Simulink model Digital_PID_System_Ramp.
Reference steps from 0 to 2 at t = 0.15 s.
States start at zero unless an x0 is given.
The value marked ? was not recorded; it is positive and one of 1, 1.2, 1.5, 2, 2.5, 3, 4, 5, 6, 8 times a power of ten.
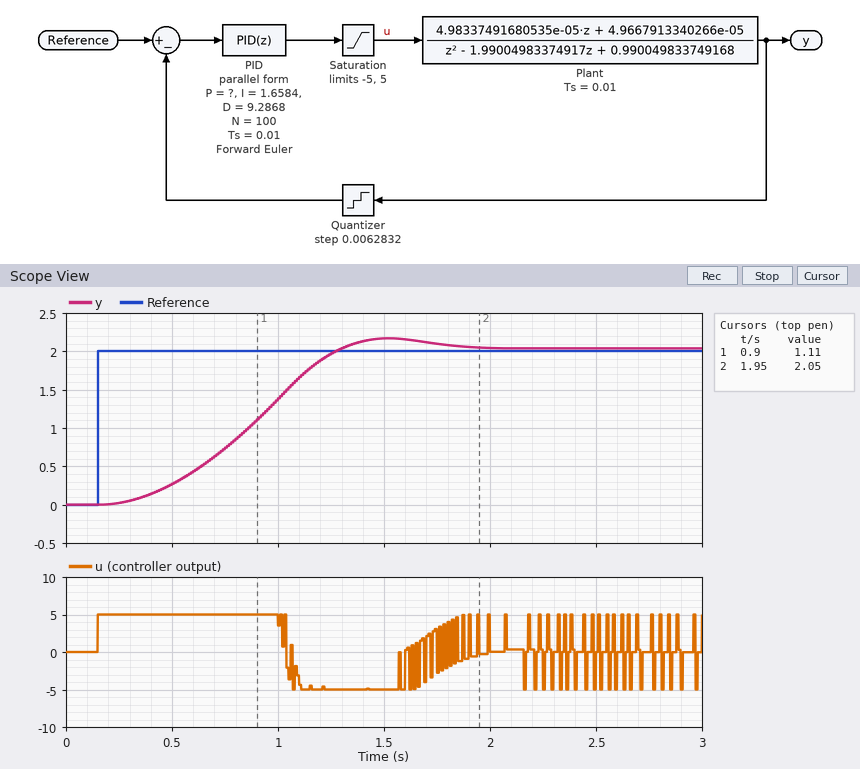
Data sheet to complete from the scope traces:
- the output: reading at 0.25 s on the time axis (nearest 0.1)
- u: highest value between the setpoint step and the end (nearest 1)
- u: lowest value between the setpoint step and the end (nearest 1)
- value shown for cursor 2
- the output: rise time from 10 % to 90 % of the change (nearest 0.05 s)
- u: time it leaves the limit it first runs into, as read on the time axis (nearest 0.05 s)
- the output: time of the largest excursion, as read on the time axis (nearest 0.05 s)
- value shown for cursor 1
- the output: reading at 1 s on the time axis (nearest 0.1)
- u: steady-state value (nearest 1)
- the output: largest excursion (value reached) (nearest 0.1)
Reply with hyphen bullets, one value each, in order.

- 0.0
- 5
- -5
- 2.05
- 0.70 s
- 1.00 s
- 1.50 s
- 1.11
- 1.4
- 0
- 2.2
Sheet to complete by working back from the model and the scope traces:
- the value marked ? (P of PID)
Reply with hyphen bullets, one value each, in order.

- 50
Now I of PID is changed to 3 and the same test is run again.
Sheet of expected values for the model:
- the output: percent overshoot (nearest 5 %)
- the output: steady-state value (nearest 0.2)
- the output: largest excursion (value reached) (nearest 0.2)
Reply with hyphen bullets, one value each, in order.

- 10 %
- 2.0
- 2.2
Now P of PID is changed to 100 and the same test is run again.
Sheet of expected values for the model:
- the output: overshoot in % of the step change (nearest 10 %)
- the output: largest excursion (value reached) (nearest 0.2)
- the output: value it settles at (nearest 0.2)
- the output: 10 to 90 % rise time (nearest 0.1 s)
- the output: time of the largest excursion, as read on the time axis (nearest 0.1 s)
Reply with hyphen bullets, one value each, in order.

- 20 %
- 2.4
- 2.0
- 0.7 s
- 1.6 s
